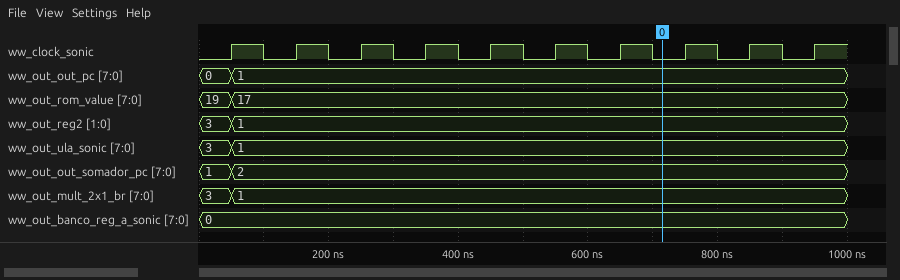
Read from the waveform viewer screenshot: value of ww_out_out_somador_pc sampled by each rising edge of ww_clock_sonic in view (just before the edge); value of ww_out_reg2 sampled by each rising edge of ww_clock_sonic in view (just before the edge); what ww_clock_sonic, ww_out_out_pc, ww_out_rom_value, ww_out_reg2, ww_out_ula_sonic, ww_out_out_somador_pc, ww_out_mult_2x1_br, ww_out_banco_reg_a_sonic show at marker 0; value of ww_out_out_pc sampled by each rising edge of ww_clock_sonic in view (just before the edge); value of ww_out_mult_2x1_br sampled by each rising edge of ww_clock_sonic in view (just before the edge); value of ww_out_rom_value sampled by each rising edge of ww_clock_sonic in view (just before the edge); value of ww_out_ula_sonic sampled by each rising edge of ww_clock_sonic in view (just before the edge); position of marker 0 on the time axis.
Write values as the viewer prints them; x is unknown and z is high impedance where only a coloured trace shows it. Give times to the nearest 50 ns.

1, 2, 2, 2, 2, 2, 2, 2, 2, 2
3, 1, 1, 1, 1, 1, 1, 1, 1, 1
ww_clock_sonic=0, ww_out_out_pc=1, ww_out_rom_value=17, ww_out_reg2=1, ww_out_ula_sonic=1, ww_out_out_somador_pc=2, ww_out_mult_2x1_br=1, ww_out_banco_reg_a_sonic=0
0, 1, 1, 1, 1, 1, 1, 1, 1, 1
3, 1, 1, 1, 1, 1, 1, 1, 1, 1
19, 17, 17, 17, 17, 17, 17, 17, 17, 17
3, 1, 1, 1, 1, 1, 1, 1, 1, 1
700 ns
